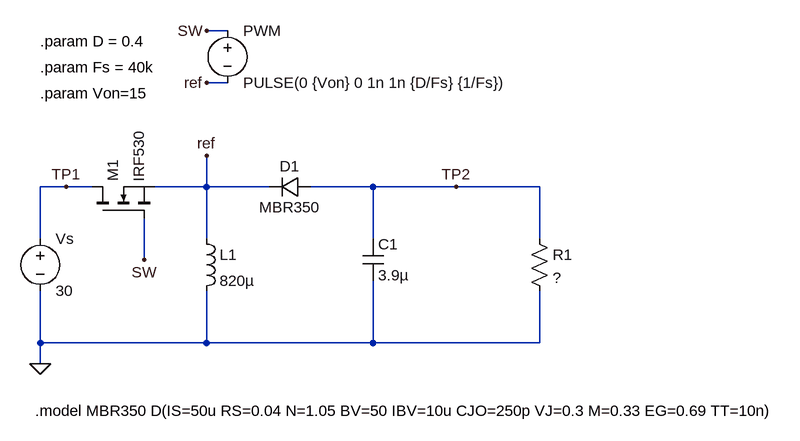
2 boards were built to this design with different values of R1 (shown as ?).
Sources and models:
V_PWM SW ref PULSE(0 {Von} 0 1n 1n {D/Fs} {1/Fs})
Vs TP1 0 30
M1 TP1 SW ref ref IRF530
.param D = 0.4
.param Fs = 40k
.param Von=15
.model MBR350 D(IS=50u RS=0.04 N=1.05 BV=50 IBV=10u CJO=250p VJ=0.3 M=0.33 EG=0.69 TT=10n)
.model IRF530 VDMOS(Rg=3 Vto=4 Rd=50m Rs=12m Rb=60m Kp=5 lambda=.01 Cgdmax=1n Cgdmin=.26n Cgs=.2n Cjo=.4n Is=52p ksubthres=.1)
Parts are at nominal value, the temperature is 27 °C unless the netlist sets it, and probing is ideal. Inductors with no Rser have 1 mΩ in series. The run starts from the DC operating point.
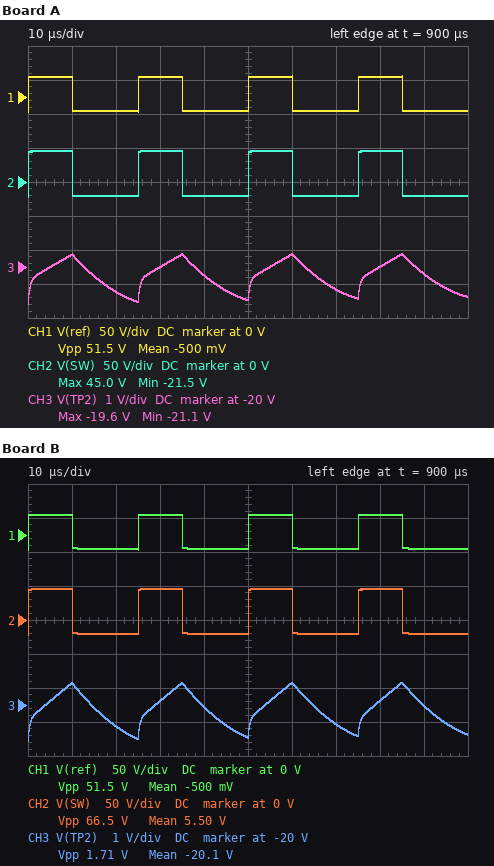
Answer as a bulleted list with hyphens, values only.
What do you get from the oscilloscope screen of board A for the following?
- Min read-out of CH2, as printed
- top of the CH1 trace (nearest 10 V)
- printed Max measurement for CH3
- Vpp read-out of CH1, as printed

- -21.5 V
- 30 V
- -19.6 V
- 51.5 V
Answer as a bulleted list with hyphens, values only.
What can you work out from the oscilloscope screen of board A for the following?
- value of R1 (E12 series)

- 68 Ω
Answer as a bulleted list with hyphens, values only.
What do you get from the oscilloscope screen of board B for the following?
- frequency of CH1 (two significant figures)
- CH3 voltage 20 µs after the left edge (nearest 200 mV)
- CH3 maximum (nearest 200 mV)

- 40 kHz
- -20.6 V
- -19.4 V
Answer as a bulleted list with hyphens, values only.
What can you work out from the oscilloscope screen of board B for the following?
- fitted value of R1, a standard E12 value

- 47 Ω
